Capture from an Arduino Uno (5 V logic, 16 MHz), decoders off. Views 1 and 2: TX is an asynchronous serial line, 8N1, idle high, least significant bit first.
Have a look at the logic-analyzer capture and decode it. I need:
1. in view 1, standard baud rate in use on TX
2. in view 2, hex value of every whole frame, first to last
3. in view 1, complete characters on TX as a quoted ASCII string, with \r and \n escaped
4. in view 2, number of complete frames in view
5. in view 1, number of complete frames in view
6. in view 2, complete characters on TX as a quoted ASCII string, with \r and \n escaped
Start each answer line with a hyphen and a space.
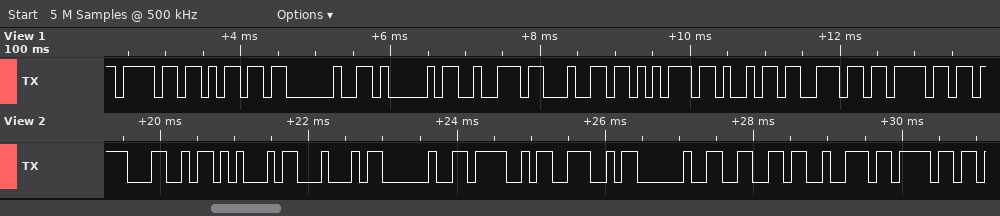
- 9600 baud
- 0x4C 0x45 0x44 0x20 0x4F 0x4E 0x20 0x66 0x72 0x6F
- "om Arduino"
- 10
- 10
- "LED ON fro"
